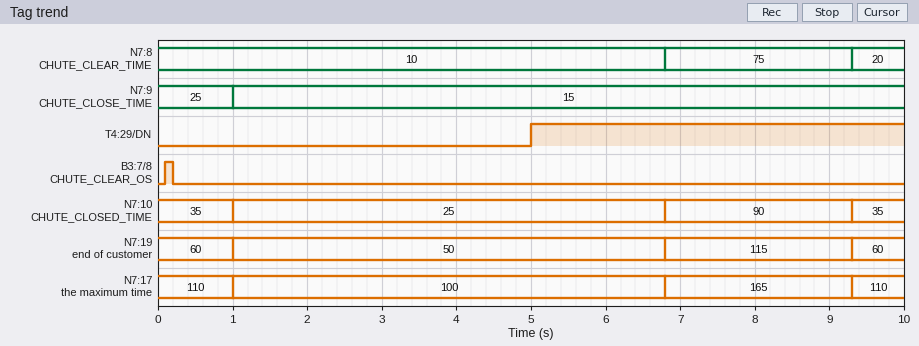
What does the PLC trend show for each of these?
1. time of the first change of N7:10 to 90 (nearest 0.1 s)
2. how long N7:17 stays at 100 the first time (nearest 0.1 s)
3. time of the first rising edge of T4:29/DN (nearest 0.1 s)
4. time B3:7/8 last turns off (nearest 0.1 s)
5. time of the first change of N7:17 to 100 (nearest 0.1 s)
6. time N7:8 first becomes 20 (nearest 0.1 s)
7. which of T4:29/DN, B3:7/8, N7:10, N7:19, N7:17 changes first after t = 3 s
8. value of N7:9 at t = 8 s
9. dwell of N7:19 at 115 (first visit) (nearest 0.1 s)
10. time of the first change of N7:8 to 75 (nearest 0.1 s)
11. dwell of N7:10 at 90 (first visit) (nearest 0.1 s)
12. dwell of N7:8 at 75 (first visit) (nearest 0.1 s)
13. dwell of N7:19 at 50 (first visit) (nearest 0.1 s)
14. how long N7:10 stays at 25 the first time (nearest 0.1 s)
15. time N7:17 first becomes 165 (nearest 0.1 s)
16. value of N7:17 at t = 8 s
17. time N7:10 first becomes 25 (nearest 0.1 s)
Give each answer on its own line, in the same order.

6.8 s
5.8 s
5.0 s
0.2 s
1.0 s
9.3 s
T4:29/DN
15
2.5 s
6.8 s
2.5 s
2.5 s
5.8 s
5.8 s
6.8 s
165
1.0 s
